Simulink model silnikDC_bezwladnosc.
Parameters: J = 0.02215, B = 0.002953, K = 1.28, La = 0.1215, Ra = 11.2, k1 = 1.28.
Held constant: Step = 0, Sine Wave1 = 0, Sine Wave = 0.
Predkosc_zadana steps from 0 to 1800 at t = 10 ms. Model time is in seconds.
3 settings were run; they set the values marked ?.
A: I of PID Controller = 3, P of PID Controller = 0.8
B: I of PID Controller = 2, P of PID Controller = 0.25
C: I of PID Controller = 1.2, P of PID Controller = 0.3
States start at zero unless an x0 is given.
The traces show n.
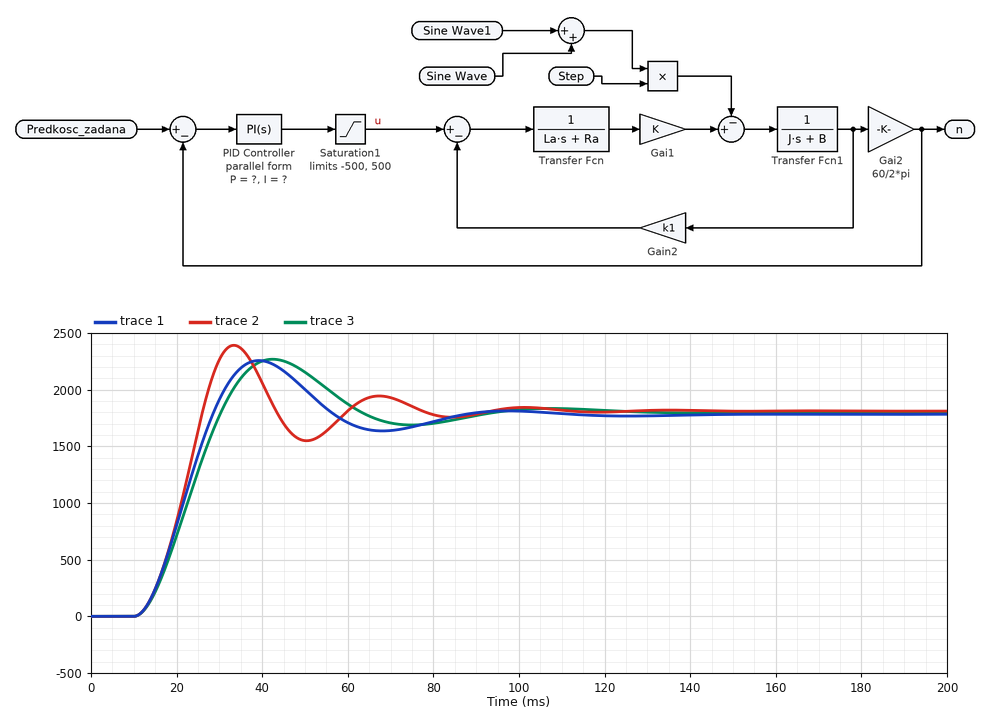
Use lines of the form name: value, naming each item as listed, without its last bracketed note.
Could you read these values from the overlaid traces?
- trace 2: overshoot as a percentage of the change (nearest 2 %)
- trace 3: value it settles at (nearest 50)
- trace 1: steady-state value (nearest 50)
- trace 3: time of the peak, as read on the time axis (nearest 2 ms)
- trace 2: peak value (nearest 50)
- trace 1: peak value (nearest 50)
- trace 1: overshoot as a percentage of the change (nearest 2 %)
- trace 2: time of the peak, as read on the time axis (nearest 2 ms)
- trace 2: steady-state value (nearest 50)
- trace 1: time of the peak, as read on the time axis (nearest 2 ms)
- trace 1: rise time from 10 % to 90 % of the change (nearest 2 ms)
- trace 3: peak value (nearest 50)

trace 2: overshoot as a percentage of the change: 32 %
trace 3: value it settles at: 1800
trace 1: steady-state value: 1800
trace 3: time of the peak, as read on the time axis: 42 ms
trace 2: peak value: 2400
trace 1: peak value: 2250
trace 1: overshoot as a percentage of the change: 26 %
trace 2: time of the peak, as read on the time axis: 34 ms
trace 2: steady-state value: 1800
trace 1: time of the peak, as read on the time axis: 40 ms
trace 1: rise time from 10 % to 90 % of the change: 12 ms
trace 3: peak value: 2250
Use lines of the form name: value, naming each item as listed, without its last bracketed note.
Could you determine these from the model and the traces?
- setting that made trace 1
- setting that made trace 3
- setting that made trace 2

setting that made trace 1: C
setting that made trace 3: B
setting that made trace 2: A
